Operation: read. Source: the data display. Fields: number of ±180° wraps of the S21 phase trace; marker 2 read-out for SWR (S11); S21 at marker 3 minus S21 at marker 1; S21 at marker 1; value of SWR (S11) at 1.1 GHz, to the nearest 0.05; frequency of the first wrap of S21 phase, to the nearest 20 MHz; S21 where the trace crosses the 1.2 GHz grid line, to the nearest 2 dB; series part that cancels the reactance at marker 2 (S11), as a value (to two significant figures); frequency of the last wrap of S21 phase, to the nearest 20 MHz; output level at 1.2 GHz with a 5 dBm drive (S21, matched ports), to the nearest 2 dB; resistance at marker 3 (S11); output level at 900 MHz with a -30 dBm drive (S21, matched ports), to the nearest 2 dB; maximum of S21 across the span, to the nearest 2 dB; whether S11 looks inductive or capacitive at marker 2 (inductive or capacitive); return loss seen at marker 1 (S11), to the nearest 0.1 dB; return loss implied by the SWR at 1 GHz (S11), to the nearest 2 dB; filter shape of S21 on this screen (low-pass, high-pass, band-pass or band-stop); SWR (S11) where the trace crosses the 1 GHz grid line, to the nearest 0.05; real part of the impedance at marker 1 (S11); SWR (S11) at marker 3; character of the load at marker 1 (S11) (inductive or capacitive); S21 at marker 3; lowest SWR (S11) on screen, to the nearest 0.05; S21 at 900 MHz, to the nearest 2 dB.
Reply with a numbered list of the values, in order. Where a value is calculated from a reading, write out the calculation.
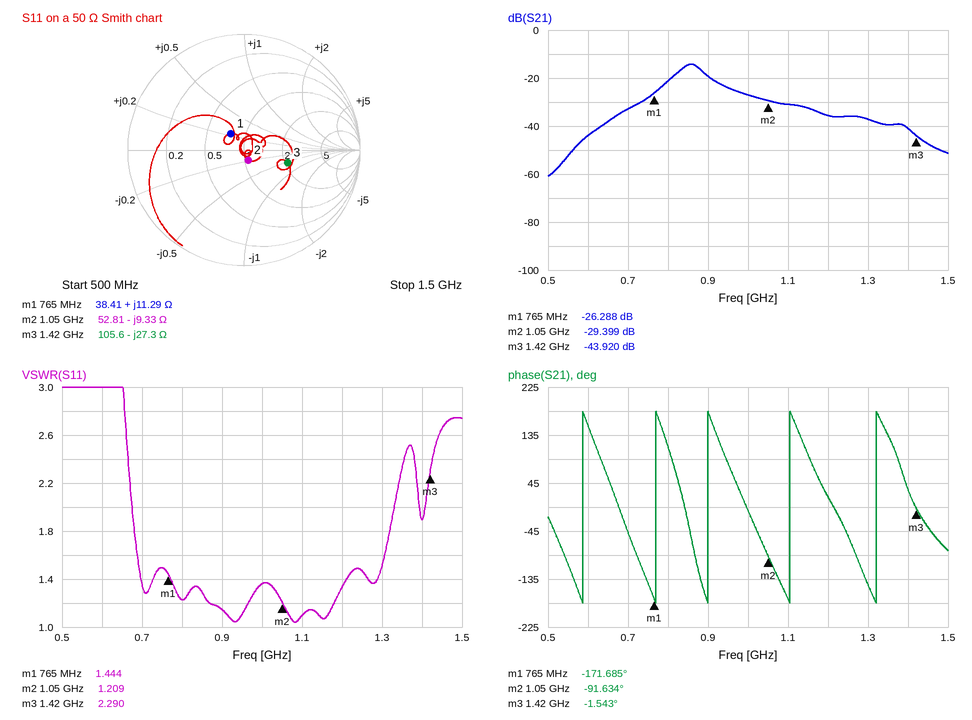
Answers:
1. 5
2. 1.209
3. -43.92 − (-26.288) = -17.632 dB
4. -26.288 dB
5. 1.10
6. 580 MHz
7. -36 dB
8. L = 9.33 Ω/(2π × 1.05 GHz) ≈ 1.4 nH
9. 1.32 GHz
10. 5 dBm + (-36 dB) = -30 dBm
11. 105.6 Ω
12. -30 dBm + (-20 dB) = -50 dBm
13. -14 dB
14. capacitive
15. 14.8 dB
16. −20 log10((1.35 − 1)/(1.35 + 1)) ≈ 16 dB
17. band-pass
18. 1.35
19. 38.41 Ω
20. 2.290
21. inductive
22. -43.920 dB
23. 1.05
24. -20 dB
